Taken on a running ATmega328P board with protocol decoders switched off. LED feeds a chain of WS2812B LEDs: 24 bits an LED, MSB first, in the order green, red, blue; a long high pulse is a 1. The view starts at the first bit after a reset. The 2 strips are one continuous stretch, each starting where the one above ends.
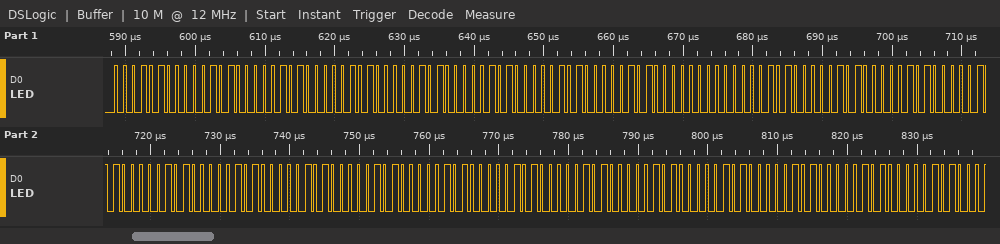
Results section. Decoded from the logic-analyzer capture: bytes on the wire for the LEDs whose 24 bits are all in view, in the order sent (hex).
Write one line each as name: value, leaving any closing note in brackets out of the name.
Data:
bytes on the wire for the LEDs whose 24 bits are all in view, in the order sent: 14 14 14 14 14 14 14 14 00 14 14 14 14 14 14 14 14 14 14 14 14 14 14 14
